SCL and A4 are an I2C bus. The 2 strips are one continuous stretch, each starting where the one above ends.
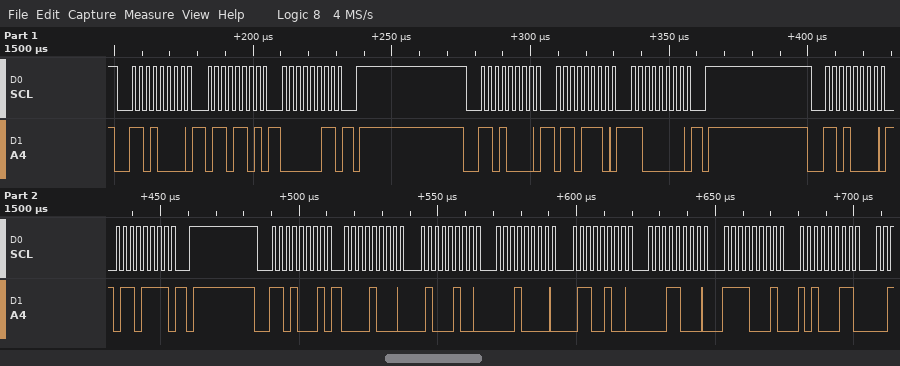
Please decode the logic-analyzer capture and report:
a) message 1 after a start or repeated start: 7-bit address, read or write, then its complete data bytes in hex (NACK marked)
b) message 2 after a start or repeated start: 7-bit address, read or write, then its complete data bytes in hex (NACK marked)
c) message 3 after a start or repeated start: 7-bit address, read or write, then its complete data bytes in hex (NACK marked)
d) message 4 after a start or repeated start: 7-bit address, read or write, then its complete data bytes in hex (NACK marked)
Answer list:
0x68 write: 6D 03
0x68 write: 6E C0
0x68 write: 6F
0x68 read: 08 44 10 64 18 F1 A3
